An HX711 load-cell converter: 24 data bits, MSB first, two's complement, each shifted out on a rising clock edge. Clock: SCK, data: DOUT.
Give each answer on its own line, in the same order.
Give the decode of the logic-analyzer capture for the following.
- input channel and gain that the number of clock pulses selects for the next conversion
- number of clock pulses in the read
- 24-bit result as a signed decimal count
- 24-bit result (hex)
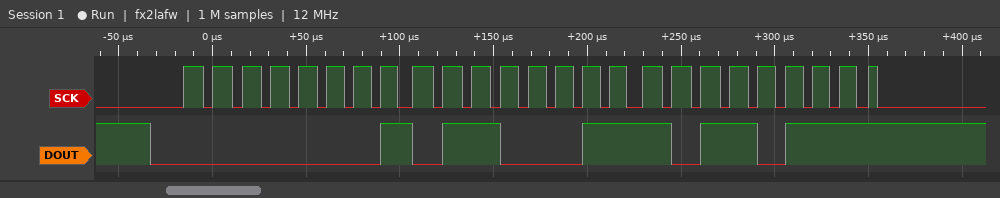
channel A, gain 128
25
91063
0x0163B7
